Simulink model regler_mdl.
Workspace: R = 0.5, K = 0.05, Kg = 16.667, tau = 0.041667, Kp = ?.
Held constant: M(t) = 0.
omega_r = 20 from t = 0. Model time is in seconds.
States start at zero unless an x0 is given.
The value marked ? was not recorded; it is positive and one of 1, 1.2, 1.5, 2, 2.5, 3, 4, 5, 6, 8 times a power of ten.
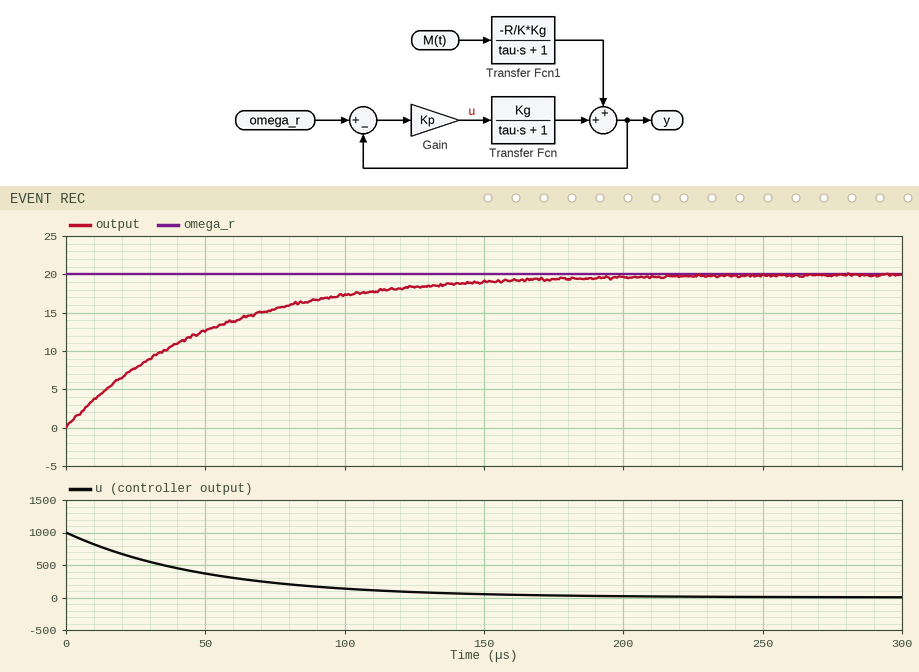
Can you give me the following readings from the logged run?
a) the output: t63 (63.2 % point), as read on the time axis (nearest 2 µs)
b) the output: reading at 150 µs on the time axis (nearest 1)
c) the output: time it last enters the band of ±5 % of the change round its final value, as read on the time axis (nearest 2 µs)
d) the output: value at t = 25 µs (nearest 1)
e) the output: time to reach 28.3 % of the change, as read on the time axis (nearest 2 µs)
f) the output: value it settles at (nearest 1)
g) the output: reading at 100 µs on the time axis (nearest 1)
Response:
50 µs
19
150 µs
8
16 µs
20
17
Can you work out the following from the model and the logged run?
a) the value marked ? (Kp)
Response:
50
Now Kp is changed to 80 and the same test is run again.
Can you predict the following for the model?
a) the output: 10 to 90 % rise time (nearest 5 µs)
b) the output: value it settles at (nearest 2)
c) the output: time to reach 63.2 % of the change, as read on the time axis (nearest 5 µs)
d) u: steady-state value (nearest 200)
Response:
70 µs
20
30 µs
0
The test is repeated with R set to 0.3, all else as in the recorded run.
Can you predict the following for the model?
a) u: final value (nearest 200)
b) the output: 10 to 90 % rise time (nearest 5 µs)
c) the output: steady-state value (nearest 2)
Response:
0
110 µs
20
